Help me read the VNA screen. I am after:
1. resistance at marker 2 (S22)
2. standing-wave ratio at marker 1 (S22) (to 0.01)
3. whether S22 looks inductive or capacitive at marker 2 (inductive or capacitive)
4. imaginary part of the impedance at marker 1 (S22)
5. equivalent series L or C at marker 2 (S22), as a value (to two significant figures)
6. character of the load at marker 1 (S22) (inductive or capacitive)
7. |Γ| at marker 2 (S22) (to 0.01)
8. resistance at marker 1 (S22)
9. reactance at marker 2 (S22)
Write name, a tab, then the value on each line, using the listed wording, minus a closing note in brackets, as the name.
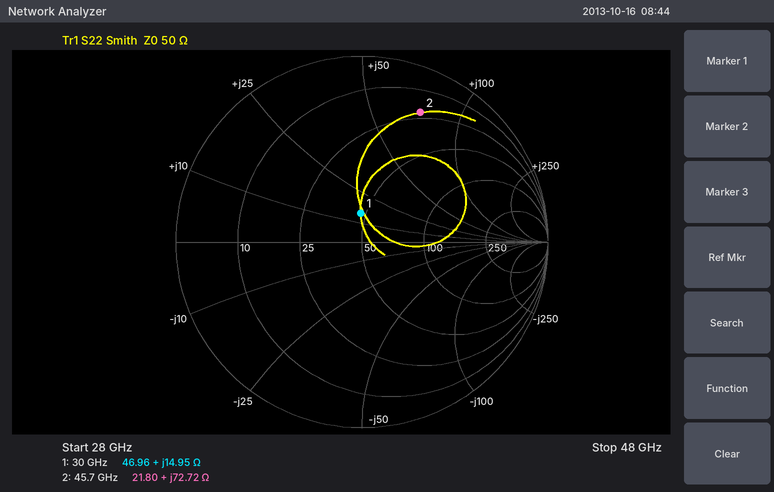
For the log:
resistance at marker 2	21.80 Ω
standing-wave ratio at marker 1 (S22)	1.37
whether S22 looks inductive or capacitive at marker 2	inductive
imaginary part of the impedance at marker 1	+14.95 Ω
equivalent series L or C at marker 2 (S22), as a value	250 pH
character of the load at marker 1 (S22)	inductive
|Γ| at marker 2 (S22)	0.76
resistance at marker 1	46.96 Ω
reactance at marker 2	+72.72 Ω
